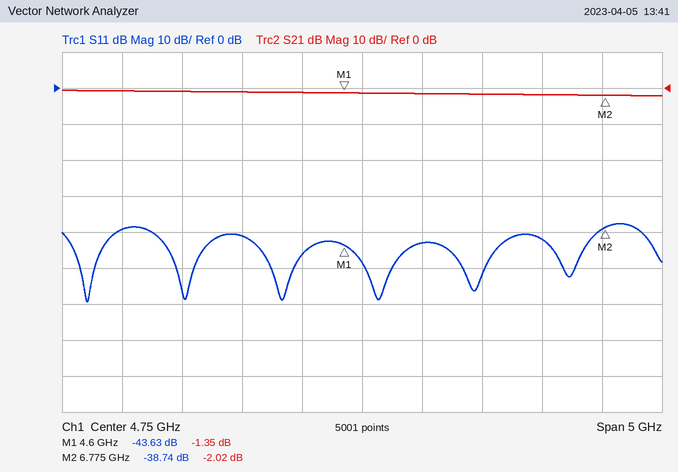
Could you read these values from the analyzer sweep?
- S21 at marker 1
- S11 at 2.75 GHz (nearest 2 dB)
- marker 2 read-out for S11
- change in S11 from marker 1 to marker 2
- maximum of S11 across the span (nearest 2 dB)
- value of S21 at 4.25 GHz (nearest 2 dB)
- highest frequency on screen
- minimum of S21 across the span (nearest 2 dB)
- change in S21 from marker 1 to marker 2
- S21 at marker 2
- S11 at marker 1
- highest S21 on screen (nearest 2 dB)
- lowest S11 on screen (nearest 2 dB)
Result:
-1.35 dB
-40 dB
-38.74 dB
4.89 dB
-38 dB
-2 dB
7.25 GHz
-2 dB
-0.67 dB
-2.02 dB
-43.63 dB
0 dB
-60 dB
